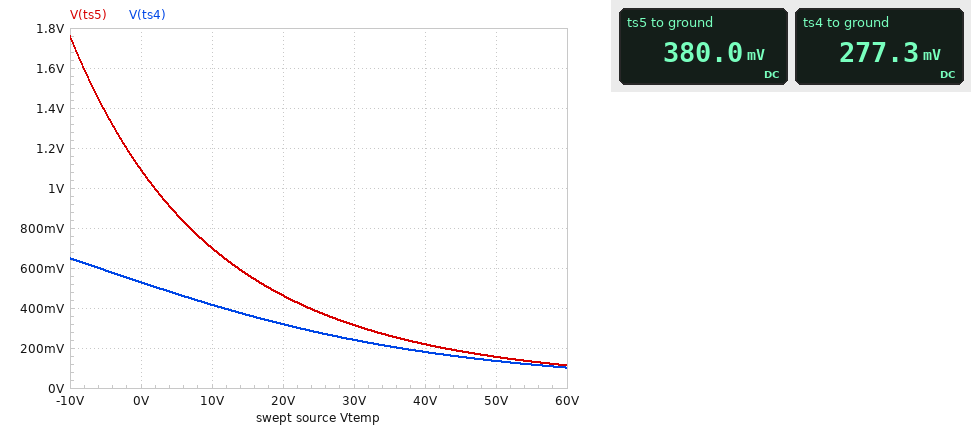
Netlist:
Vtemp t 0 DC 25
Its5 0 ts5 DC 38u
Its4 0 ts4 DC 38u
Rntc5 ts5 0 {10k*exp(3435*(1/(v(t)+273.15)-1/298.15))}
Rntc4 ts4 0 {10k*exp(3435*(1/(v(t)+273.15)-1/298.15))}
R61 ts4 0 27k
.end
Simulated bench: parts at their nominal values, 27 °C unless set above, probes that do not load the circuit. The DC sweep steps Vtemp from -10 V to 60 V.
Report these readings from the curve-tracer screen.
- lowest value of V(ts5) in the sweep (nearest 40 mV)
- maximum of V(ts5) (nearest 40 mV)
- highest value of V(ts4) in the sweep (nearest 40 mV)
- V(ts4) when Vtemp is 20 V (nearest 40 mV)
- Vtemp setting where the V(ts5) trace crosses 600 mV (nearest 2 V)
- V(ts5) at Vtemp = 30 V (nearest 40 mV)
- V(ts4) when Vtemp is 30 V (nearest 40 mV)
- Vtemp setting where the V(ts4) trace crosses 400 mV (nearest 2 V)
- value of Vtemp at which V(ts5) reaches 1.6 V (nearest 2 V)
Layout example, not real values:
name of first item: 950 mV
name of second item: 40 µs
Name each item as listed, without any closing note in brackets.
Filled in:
lowest value of V(ts5) in the sweep: 120 mV
maximum of V(ts5): 1.76 V
highest value of V(ts4) in the sweep: 640 mV
V(ts4) when Vtemp is 20 V: 320 mV
Vtemp setting where the V(ts5) trace crosses 600 mV: 14 V
V(ts5) at Vtemp = 30 V: 320 mV
V(ts4) when Vtemp is 30 V: 240 mV
Vtemp setting where the V(ts4) trace crosses 400 mV: 12 V
value of Vtemp at which V(ts5) reaches 1.6 V: -8 V
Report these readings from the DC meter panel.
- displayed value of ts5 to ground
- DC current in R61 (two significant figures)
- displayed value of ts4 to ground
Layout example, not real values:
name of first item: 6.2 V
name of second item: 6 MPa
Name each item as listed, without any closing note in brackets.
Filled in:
displayed value of ts5 to ground: 380.0 mV
DC current in R61: 10 µA
displayed value of ts4 to ground: 277.3 mV
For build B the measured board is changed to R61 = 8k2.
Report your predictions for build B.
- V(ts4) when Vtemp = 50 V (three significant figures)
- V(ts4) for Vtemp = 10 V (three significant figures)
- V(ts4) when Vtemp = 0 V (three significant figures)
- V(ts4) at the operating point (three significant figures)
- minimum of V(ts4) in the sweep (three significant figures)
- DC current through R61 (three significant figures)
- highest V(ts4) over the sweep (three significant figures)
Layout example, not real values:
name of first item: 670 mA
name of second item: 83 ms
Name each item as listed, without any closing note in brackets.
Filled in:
V(ts4) when Vtemp = 50 V: 104 mV
V(ts4) for Vtemp = 10 V: 216 mV
V(ts4) when Vtemp = 0 V: 242 mV
V(ts4) at the operating point: 171 mV
minimum of V(ts4) in the sweep: 83.1 mV
DC current through R61: 20.9 µA
highest V(ts4) over the sweep: 265 mV
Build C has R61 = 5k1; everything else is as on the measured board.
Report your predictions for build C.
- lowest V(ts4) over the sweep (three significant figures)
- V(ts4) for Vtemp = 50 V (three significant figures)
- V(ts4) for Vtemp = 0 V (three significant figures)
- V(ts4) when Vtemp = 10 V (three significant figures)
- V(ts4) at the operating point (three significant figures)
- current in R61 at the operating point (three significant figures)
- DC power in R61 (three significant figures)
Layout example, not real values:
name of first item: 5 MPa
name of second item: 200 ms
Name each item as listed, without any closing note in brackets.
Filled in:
lowest V(ts4) over the sweep: 71.5 mV
V(ts4) for Vtemp = 50 V: 86.4 mV
V(ts4) for Vtemp = 0 V: 165 mV
V(ts4) when Vtemp = 10 V: 152 mV
V(ts4) at the operating point: 128 mV
current in R61 at the operating point: 25.2 µA
DC power in R61: 3.23 µW
